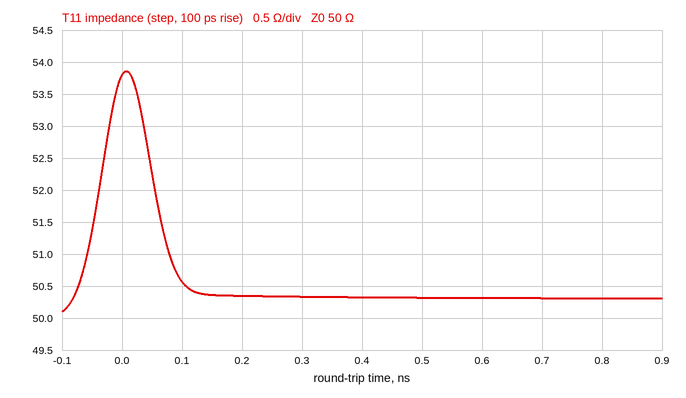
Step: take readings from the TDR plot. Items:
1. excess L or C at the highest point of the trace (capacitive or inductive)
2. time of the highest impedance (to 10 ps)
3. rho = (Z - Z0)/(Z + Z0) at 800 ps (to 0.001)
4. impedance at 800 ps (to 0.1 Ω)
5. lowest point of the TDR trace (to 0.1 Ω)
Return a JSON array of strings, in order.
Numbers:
["inductive", "10 ps", "+0.003", "50.3 Ω", "50.1 Ω"]
